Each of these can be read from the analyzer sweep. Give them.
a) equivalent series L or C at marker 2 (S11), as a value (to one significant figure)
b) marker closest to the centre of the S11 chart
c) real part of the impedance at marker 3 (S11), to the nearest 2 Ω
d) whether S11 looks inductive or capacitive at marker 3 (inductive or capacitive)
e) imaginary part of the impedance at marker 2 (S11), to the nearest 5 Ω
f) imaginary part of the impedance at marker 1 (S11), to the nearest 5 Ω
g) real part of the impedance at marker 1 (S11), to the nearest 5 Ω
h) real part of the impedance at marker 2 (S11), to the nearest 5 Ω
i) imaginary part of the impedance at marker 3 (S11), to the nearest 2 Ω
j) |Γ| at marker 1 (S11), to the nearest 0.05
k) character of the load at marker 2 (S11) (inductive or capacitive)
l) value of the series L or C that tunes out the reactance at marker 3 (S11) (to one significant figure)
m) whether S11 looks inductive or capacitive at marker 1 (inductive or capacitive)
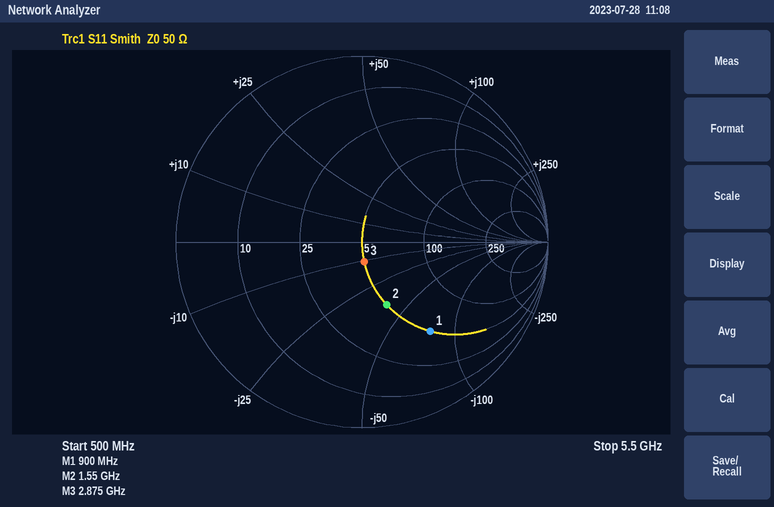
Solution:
3 pF
marker 3
50 Ω
capacitive
-40 Ω
-75 Ω
50 Ω
50 Ω
-10 Ω
0.60
capacitive
600 pH
capacitive
